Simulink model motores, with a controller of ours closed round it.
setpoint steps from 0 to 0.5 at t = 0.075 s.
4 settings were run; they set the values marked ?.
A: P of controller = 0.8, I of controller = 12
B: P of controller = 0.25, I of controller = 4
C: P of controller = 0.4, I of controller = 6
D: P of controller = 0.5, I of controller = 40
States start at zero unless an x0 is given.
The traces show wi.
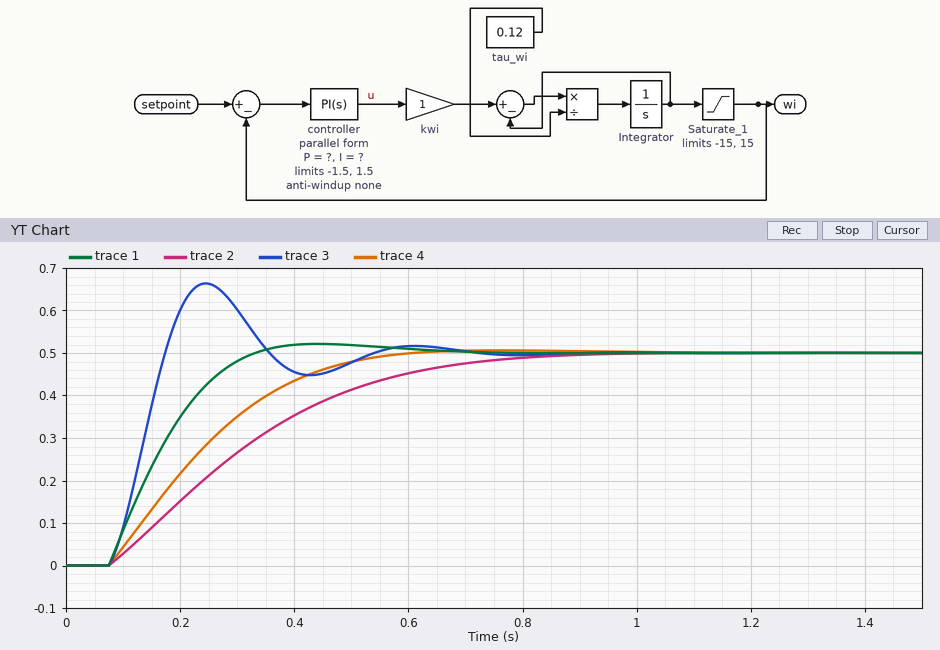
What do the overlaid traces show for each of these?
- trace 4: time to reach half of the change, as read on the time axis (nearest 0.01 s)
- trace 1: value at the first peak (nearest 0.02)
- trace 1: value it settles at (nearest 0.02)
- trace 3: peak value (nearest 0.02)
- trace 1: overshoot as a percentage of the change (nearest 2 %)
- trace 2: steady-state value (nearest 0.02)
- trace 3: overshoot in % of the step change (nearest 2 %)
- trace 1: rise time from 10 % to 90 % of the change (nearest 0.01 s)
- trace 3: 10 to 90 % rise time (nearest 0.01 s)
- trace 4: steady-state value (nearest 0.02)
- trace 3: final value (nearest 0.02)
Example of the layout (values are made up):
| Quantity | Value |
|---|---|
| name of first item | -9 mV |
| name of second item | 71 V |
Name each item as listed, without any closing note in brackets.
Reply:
| Quantity | Value |
|---|---|
| trace 4: time to reach half of the change, as read on the time axis | 0.22 s |
| trace 1: value at the first peak | 0.52 |
| trace 1: value it settles at | 0.50 |
| trace 3: peak value | 0.66 |
| trace 1: overshoot as a percentage of the change | 4 % |
| trace 2: steady-state value | 0.50 |
| trace 3: overshoot in % of the step change | 32 % |
| trace 1: rise time from 10 % to 90 % of the change | 0.18 s |
| trace 3: 10 to 90 % rise time | 0.07 s |
| trace 4: steady-state value | 0.50 |
| trace 3: final value | 0.50 |
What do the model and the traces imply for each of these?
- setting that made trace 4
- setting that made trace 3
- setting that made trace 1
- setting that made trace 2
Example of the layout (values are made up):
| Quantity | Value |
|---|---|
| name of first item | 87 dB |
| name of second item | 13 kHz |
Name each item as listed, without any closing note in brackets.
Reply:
| Quantity | Value |
|---|---|
| setting that made trace 4 | C |
| setting that made trace 3 | D |
| setting that made trace 1 | A |
| setting that made trace 2 | B |
